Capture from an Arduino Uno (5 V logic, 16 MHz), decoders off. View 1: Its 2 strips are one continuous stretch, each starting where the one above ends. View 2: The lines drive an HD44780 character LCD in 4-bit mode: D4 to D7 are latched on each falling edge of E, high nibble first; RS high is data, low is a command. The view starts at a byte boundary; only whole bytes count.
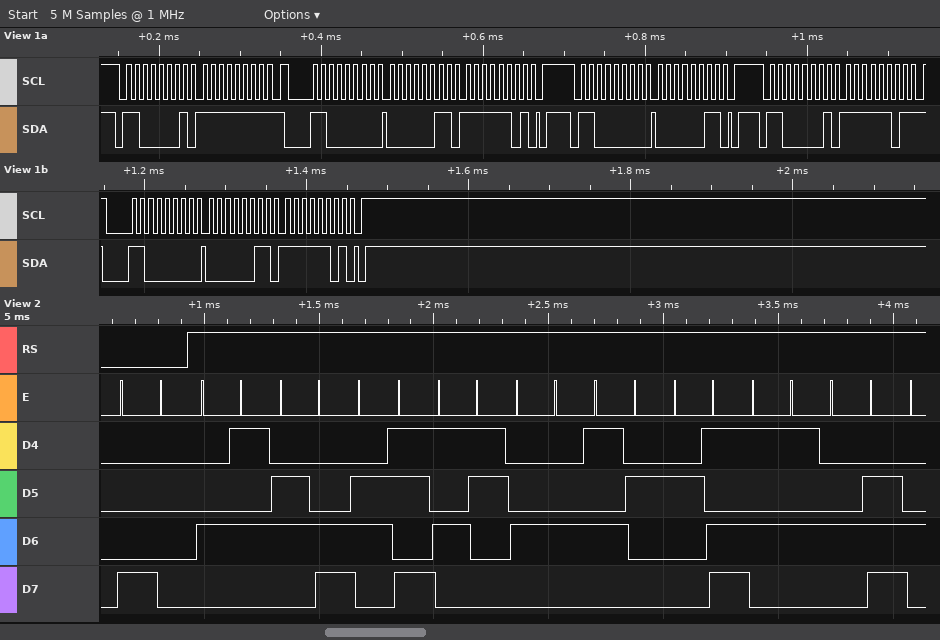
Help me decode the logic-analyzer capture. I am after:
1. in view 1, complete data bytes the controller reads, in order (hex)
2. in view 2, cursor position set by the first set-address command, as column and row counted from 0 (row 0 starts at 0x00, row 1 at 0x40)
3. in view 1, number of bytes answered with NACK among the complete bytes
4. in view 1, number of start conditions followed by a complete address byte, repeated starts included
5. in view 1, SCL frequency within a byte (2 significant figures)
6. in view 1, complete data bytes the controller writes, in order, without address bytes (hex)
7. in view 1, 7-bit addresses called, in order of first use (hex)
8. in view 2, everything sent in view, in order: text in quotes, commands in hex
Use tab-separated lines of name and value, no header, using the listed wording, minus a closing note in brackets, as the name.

in view 1, complete data bytes the controller reads, in order	FF FD
in view 2, cursor position set by the first set-address command, as column and row counted from 0	column 0, row 0
in view 1, number of bytes answered with NACK among the complete bytes	2
in view 1, number of start conditions followed by a complete address byte, repeated starts included	5
in view 1, SCL frequency within a byte	100 kHz
in view 1, complete data bytes the controller writes, in order, without address bytes	03 FD 03 03 FD
in view 1, 7-bit addresses called, in order of first use	0x60
in view 2, everything sent in view, in order: text in quotes, commands in hex	0x80 "ElkSDR-UN"
